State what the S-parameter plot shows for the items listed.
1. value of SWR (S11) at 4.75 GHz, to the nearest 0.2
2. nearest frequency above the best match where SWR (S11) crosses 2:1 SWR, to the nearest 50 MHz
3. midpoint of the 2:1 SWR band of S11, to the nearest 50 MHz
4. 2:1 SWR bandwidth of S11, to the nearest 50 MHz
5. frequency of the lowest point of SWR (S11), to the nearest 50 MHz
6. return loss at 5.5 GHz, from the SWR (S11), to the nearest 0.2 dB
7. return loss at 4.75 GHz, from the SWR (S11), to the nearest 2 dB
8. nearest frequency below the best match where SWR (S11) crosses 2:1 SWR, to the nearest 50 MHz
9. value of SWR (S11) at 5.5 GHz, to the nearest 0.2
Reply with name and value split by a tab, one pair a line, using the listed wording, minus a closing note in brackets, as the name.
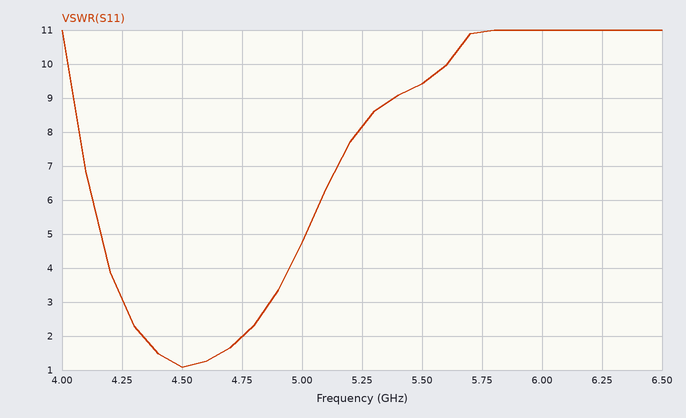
value of SWR (S11) at 4.75 GHz, to the nearest 0.2	2.0
nearest frequency above the best match where SWR (S11) crosses 2:1 SWR, to the nearest 50 MHz	4.75 GHz
midpoint of the 2:1 SWR band of S11, to the nearest 50 MHz	4.55 GHz
2:1 SWR bandwidth of S11, to the nearest 50 MHz	400 MHz
frequency of the lowest point of SWR (S11), to the nearest 50 MHz	4.50 GHz
return loss at 5.5 GHz, from the SWR (S11), to the nearest 0.2 dB	1.8 dB
return loss at 4.75 GHz, from the SWR (S11), to the nearest 2 dB	10 dB
nearest frequency below the best match where SWR (S11) crosses 2:1 SWR, to the nearest 50 MHz	4.35 GHz
value of SWR (S11) at 5.5 GHz, to the nearest 0.2	9.4
